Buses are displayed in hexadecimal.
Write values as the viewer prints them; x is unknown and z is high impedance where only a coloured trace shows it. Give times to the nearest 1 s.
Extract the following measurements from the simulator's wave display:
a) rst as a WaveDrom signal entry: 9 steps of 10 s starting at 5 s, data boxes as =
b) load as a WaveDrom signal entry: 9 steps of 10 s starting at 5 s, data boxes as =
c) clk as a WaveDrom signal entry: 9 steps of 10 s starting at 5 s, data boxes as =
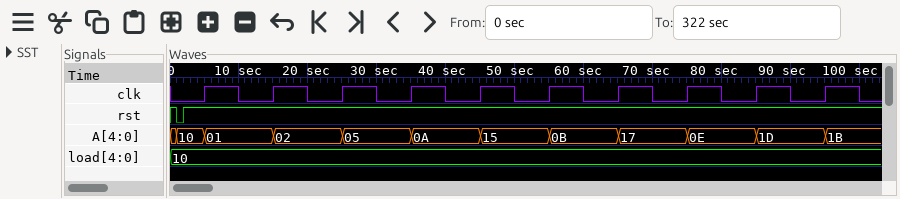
{name: 'rst', wave: '1........'}
{name: 'load', wave: '=........', data: '10'}
{name: 'clk', wave: 'p........'}
